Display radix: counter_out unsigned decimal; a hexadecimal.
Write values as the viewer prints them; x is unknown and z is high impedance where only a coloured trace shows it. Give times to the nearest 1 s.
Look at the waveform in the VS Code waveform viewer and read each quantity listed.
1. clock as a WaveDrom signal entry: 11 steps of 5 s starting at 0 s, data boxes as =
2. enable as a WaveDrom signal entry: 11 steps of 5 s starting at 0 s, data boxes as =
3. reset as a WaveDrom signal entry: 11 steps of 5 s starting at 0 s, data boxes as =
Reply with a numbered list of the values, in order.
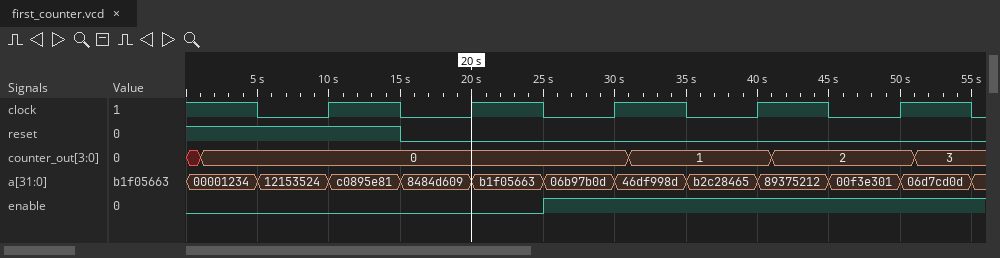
1. {name: 'clock', wave: '10101010101'}
2. {name: 'enable', wave: '0....1.....'}
3. {name: 'reset', wave: '1..0.......'}
